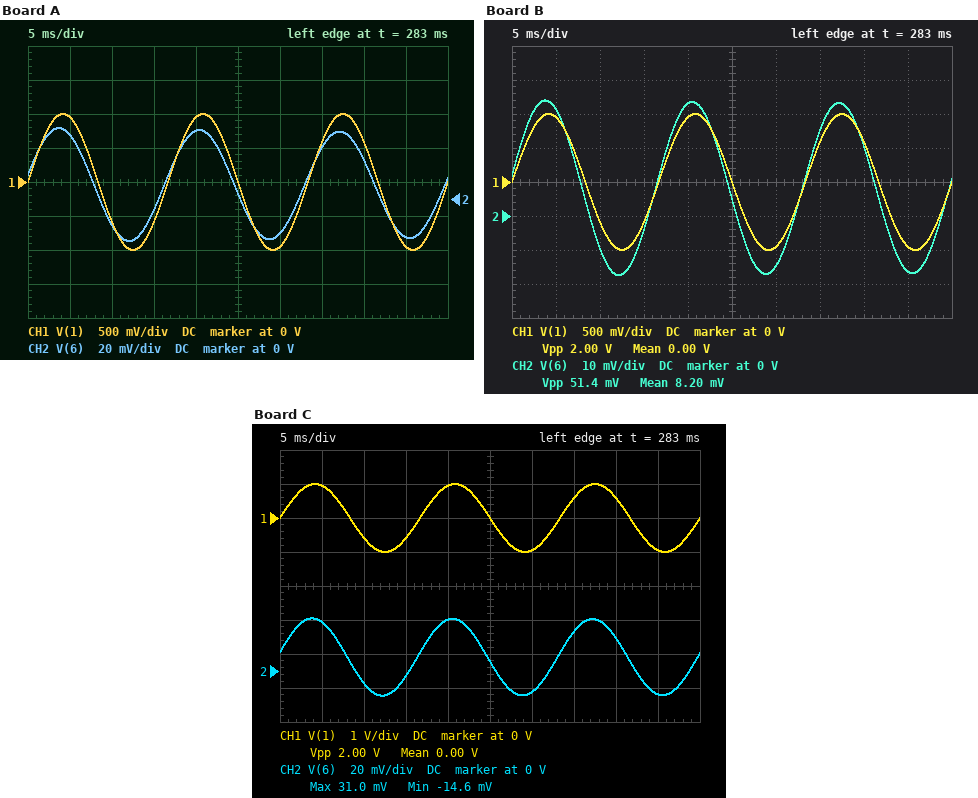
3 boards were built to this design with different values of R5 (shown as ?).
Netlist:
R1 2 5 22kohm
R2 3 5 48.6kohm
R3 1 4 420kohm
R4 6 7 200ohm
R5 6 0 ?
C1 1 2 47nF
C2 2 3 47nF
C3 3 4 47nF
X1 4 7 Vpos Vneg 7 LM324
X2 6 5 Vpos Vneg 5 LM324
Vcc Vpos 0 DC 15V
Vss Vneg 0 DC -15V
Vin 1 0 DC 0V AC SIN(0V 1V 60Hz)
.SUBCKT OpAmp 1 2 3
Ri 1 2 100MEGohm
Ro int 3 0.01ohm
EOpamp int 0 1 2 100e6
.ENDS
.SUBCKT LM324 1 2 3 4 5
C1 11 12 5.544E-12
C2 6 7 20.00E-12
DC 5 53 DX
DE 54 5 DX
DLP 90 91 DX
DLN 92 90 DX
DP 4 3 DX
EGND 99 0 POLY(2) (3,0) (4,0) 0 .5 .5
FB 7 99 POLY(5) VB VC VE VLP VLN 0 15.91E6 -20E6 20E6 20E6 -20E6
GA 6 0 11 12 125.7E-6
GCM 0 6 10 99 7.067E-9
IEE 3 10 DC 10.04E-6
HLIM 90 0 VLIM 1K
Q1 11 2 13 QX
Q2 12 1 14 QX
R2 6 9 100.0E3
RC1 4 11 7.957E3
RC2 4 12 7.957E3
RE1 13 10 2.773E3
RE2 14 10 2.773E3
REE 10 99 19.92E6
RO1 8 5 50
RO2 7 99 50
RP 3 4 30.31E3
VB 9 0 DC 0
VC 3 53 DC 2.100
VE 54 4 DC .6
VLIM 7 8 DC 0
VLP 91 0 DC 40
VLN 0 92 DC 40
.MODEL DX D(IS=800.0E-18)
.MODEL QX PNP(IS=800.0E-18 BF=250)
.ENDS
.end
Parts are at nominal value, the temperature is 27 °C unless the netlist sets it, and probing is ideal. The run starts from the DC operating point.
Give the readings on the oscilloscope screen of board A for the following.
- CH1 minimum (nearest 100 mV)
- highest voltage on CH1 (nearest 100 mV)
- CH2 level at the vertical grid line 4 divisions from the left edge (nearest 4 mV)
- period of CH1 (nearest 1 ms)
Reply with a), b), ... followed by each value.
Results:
a) -1.0 V
b) 1.0 V
c) 40 mV
d) 17 ms
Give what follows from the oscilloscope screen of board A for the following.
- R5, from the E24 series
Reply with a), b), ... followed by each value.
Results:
a) 11 kΩ
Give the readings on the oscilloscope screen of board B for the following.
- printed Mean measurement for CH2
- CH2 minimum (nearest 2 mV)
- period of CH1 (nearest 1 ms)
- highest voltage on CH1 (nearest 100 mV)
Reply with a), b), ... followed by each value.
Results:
a) 8.20 mV
b) -18 mV
c) 17 ms
d) 1.0 V
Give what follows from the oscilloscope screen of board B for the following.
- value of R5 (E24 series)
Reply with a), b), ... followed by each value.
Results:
a) 9.1 kΩ
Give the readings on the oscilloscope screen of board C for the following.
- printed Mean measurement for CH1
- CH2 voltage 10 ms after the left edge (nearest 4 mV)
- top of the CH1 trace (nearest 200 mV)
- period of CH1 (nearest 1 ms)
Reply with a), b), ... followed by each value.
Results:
a) 0.00 V
b) -8 mV
c) 1.0 V
d) 17 ms
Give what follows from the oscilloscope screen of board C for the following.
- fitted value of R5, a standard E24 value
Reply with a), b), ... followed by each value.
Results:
a) 8.2 kΩ
